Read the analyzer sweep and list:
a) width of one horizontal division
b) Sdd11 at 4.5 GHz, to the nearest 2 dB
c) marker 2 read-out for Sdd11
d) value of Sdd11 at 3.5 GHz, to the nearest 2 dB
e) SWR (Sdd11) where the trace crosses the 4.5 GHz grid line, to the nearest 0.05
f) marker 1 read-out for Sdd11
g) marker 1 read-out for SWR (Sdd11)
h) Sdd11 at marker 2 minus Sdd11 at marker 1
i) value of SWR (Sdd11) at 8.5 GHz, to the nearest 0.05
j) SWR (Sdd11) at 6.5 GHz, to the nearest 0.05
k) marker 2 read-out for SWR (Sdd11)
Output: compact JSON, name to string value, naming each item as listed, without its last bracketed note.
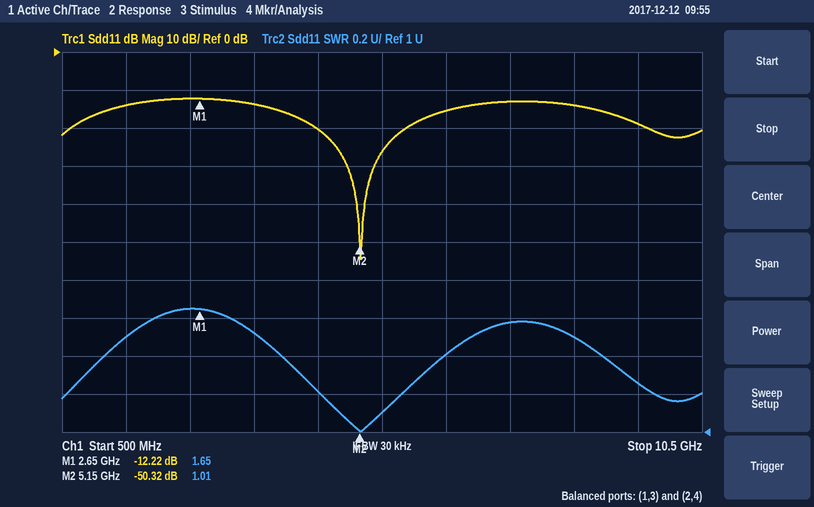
{"width of one horizontal division": "1 GHz", "Sdd11 at 4.5 GHz, to the nearest 2 dB": "-20 dB", "marker 2 read-out for Sdd11": "-50.32 dB", "value of Sdd11 at 3.5 GHz, to the nearest 2 dB": "-14 dB", "SWR (Sdd11) where the trace crosses the 4.5 GHz grid line, to the nearest 0.05": "1.20", "marker 1 read-out for Sdd11": "-12.22 dB", "marker 1 read-out for SWR": "1.65", "Sdd11 at marker 2 minus Sdd11 at marker 1": "-38.10 dB", "value of SWR (Sdd11) at 8.5 GHz, to the nearest 0.05": "1.50", "SWR (Sdd11) at 6.5 GHz, to the nearest 0.05": "1.40", "marker 2 read-out for SWR": "1.01"}
